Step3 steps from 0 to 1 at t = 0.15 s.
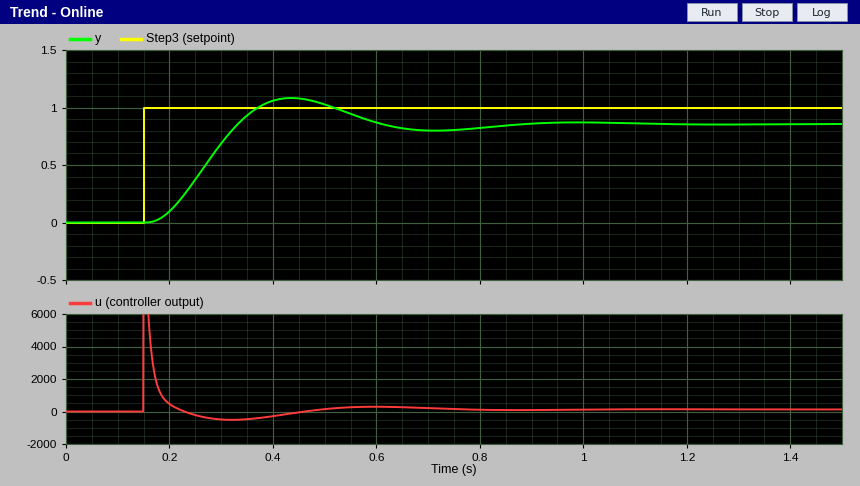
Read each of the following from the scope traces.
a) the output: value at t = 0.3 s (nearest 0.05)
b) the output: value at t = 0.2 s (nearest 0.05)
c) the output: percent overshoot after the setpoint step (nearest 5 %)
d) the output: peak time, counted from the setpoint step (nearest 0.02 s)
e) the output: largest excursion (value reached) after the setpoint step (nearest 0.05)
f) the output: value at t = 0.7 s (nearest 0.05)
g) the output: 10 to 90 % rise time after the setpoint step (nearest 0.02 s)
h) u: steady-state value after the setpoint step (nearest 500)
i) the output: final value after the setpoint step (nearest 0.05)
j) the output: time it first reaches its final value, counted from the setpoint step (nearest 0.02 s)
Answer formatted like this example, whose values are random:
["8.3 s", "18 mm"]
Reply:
["0.70", "0.10", "25 %", "0.28 s", "1.10", "0.80", "0.12 s", "0", "0.85", "0.18 s"]
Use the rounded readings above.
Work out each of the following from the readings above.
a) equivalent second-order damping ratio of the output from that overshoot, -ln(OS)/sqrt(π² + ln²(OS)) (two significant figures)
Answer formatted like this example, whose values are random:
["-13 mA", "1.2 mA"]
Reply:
["0.40"]
